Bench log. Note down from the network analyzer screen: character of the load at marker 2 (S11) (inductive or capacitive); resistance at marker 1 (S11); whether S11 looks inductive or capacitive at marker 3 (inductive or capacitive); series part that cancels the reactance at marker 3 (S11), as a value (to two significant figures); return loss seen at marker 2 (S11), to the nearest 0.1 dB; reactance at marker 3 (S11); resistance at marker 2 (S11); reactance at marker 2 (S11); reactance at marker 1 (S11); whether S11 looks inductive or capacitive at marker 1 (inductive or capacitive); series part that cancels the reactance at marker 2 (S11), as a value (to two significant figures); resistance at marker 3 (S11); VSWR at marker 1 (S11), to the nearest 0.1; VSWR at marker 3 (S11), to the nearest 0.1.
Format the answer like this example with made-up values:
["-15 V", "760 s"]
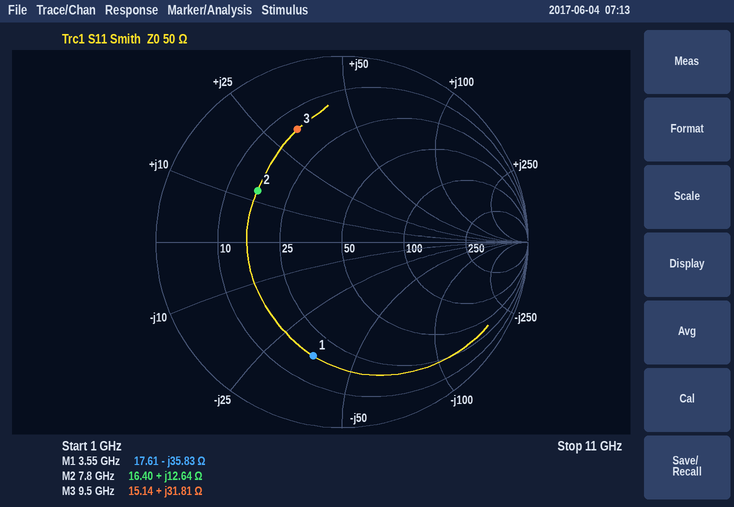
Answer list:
["inductive", "17.61 Ω", "inductive", "530 fF", "5.5 dB", "+31.81 Ω", "16.40 Ω", "+12.64 Ω", "-35.83 Ω", "capacitive", "1.6 pF", "15.14 Ω", "4.4", "4.7"]
